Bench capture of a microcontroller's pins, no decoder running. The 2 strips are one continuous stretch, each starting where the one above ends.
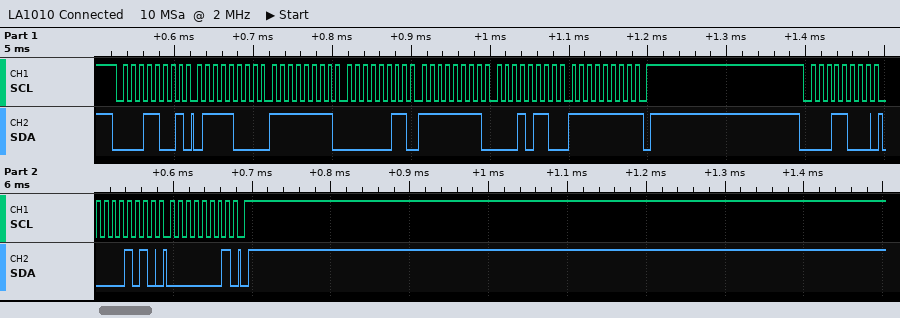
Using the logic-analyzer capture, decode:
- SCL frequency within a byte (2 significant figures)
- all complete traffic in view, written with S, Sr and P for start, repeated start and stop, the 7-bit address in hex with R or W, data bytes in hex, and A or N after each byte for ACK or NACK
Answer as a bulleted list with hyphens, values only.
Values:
- 100 kHz
- S 0CR A 78 A FF A 03 A FF A 16 A FF N P S 0CW A 0A A 01 A P
